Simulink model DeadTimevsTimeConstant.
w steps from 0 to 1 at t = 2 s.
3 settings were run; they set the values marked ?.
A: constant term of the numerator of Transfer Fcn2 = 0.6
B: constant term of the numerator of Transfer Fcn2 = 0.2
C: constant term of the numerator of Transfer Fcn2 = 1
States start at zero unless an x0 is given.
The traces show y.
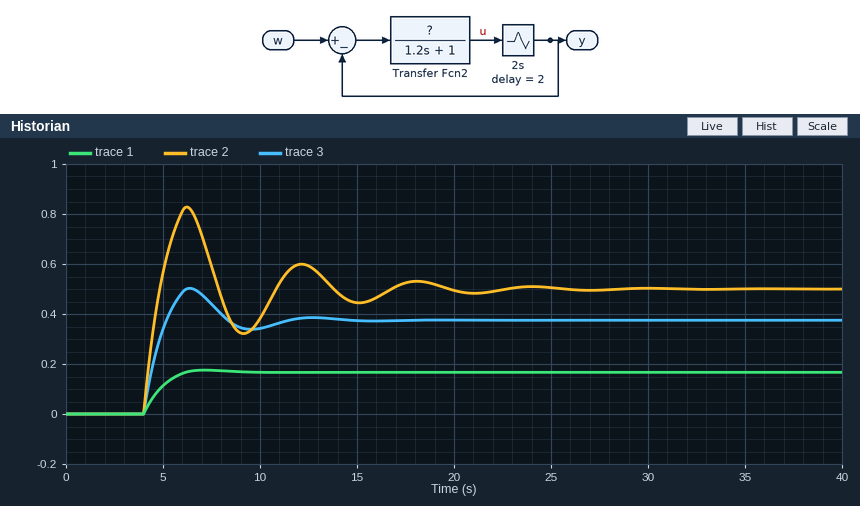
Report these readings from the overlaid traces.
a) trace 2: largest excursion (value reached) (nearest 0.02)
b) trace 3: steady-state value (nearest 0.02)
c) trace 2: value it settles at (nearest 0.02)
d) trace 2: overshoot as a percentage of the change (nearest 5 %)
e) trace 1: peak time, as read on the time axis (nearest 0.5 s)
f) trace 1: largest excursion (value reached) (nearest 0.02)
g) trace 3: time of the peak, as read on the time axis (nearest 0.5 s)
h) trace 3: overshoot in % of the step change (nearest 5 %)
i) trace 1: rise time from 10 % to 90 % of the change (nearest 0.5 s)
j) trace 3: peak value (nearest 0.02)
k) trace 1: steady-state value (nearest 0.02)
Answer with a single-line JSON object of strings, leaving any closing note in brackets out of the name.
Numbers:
{"trace 2: largest excursion (value reached)": "0.82", "trace 3: steady-state value": "0.38", "trace 2: value it settles at": "0.50", "trace 2: overshoot as a percentage of the change": "65 %", "trace 1: peak time, as read on the time axis": "7.0 s", "trace 1: largest excursion (value reached)": "0.18", "trace 3: time of the peak, as read on the time axis": "6.5 s", "trace 3: overshoot in % of the step change": "35 %", "trace 1: rise time from 10 % to 90 % of the change": "1.5 s", "trace 3: peak value": "0.50", "trace 1: steady-state value": "0.16"}
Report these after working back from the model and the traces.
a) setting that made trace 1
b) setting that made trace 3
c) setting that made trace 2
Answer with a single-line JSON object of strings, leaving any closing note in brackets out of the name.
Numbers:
{"setting that made trace 1": "B", "setting that made trace 3": "A", "setting that made trace 2": "C"}
